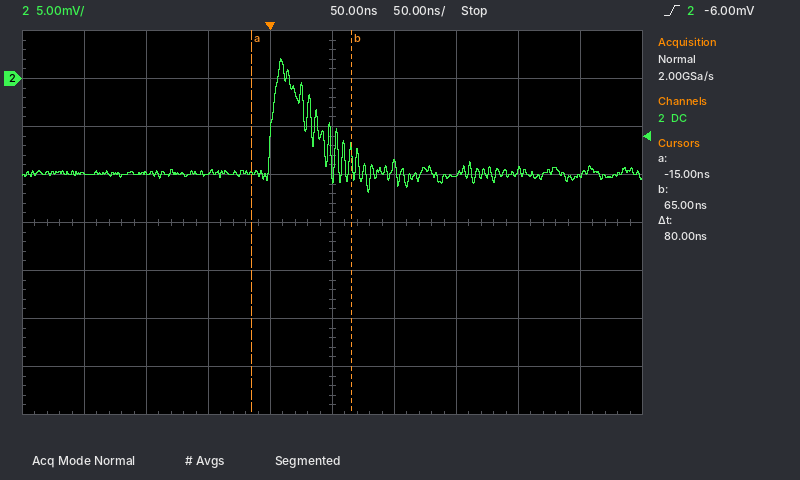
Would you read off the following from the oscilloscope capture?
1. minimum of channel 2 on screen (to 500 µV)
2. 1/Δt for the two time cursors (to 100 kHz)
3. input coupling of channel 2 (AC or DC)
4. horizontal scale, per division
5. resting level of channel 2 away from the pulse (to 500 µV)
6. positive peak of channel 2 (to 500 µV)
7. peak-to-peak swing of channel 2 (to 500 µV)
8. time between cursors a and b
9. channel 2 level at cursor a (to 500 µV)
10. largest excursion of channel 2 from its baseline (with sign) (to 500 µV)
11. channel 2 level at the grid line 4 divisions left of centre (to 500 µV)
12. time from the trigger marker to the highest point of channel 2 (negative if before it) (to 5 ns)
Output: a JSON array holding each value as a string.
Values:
["-12.0 mV", "12.5 MHz", "DC", "50 ns", "-10.0 mV", "2.0 mV", "14.0 mV", "80 ns", "-10.0 mV", "+12.0 mV", "-10.0 mV", "+10 ns"]
